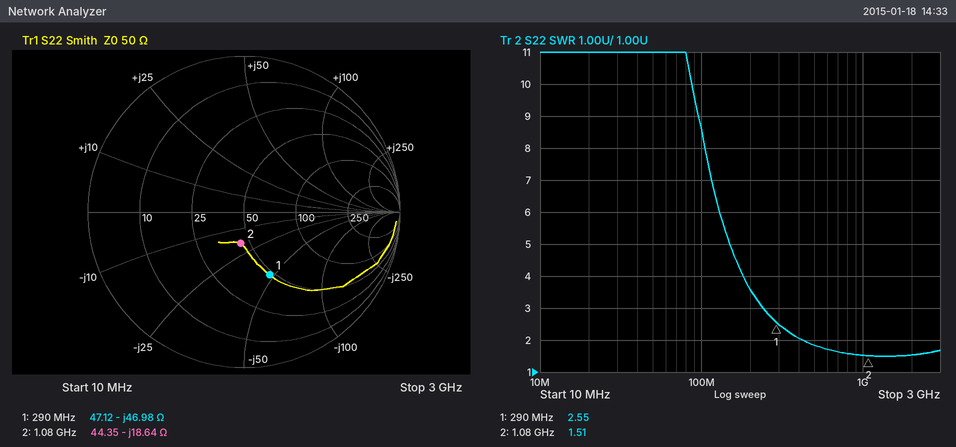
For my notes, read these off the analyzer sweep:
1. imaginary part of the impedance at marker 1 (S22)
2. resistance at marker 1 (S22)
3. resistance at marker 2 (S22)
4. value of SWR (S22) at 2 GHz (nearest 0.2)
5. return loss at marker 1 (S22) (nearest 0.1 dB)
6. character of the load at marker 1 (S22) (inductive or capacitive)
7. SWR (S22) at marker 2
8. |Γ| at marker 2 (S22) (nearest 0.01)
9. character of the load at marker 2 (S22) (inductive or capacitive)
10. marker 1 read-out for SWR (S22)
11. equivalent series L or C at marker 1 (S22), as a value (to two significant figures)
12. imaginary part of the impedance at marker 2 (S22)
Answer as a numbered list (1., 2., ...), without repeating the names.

1. -46.98 Ω
2. 47.12 Ω
3. 44.35 Ω
4. 1.6
5. 7.2 dB
6. capacitive
7. 1.51
8. 0.20
9. capacitive
10. 2.55
11. 12 pF
12. -18.64 Ω
